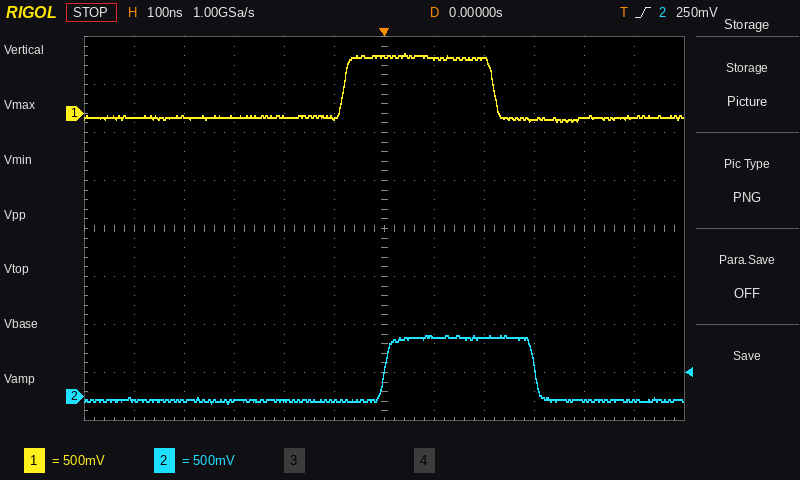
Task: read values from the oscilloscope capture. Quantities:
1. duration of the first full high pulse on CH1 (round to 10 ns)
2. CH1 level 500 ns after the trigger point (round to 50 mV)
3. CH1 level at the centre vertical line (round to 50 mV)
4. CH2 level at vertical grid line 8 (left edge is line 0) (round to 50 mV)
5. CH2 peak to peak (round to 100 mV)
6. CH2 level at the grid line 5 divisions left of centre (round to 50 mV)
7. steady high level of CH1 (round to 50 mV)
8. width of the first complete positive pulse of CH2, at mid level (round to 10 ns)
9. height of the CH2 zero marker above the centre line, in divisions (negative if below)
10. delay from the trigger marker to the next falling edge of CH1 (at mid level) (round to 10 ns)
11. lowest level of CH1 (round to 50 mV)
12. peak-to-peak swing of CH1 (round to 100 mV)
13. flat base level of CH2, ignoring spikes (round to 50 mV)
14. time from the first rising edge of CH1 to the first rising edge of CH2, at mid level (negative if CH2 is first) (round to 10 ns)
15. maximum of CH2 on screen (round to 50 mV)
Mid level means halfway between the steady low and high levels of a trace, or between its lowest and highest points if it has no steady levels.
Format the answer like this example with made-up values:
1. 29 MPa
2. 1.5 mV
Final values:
1. 300 ns
2. -50 mV
3. 600 mV
4. 600 mV
5. 700 mV
6. -50 mV
7. 600 mV
8. 300 ns
9. -3.5 div
10. 220 ns
11. -100 mV
12. 700 mV
13. -50 mV
14. +80 ns
15. 650 mV
